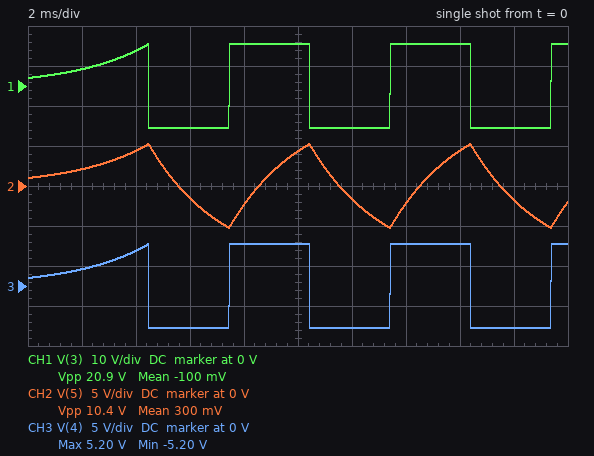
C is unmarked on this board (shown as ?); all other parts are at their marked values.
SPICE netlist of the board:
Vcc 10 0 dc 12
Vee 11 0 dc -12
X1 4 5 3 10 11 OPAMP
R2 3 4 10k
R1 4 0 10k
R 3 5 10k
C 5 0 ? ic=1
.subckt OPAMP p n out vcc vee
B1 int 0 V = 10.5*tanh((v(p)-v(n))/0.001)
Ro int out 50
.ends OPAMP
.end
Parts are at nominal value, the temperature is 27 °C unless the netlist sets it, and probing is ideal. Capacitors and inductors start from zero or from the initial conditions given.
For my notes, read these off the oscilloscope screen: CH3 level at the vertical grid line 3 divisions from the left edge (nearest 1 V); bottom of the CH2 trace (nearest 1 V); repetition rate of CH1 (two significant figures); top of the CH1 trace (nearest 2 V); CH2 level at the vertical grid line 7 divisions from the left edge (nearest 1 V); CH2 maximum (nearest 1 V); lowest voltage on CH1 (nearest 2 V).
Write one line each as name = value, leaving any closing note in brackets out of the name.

CH3 level at the vertical grid line 3 divisions from the left edge = -5 V
bottom of the CH2 trace = -5 V
repetition rate of CH1 = 170 Hz
top of the CH1 trace = 10 V
CH2 level at the vertical grid line 7 divisions from the left edge = -2 V
CH2 maximum = 5 V
lowest voltage on CH1 = -10 V
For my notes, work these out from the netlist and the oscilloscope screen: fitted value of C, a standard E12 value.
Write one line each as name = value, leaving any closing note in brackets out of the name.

fitted value of C, a standard E12 value = 270 nF
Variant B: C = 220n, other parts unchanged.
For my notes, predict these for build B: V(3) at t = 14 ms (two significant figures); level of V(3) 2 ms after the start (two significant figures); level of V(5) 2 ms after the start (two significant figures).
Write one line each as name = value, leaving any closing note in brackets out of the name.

V(3) at t = 14 ms = -10 V
level of V(3) 2 ms after the start = 5.0 V
level of V(5) 2 ms after the start = 2.5 V
